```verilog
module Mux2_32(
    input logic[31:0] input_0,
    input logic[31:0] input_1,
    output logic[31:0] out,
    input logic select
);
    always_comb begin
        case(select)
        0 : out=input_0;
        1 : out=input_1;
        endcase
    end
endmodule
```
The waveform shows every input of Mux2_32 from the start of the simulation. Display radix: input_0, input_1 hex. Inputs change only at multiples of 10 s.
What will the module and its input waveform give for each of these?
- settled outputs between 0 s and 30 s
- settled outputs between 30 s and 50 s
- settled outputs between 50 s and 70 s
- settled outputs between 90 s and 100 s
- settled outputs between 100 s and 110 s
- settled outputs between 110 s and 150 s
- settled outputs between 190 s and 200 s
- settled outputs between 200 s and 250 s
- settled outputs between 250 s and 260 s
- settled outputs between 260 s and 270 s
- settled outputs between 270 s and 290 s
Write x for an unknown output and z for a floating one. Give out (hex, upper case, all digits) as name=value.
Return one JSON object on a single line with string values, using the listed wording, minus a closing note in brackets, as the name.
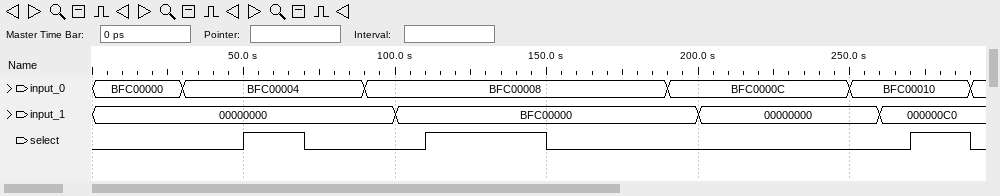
{"settled outputs between 0 s and 30 s": "out=BFC00000", "settled outputs between 30 s and 50 s": "out=BFC00004", "settled outputs between 50 s and 70 s": "out=00000000", "settled outputs between 90 s and 100 s": "out=BFC00008", "settled outputs between 100 s and 110 s": "out=BFC00008", "settled outputs between 110 s and 150 s": "out=BFC00000", "settled outputs between 190 s and 200 s": "out=BFC0000C", "settled outputs between 200 s and 250 s": "out=BFC0000C", "settled outputs between 250 s and 260 s": "out=BFC00010", "settled outputs between 260 s and 270 s": "out=BFC00010", "settled outputs between 270 s and 290 s": "out=000000C0"}
